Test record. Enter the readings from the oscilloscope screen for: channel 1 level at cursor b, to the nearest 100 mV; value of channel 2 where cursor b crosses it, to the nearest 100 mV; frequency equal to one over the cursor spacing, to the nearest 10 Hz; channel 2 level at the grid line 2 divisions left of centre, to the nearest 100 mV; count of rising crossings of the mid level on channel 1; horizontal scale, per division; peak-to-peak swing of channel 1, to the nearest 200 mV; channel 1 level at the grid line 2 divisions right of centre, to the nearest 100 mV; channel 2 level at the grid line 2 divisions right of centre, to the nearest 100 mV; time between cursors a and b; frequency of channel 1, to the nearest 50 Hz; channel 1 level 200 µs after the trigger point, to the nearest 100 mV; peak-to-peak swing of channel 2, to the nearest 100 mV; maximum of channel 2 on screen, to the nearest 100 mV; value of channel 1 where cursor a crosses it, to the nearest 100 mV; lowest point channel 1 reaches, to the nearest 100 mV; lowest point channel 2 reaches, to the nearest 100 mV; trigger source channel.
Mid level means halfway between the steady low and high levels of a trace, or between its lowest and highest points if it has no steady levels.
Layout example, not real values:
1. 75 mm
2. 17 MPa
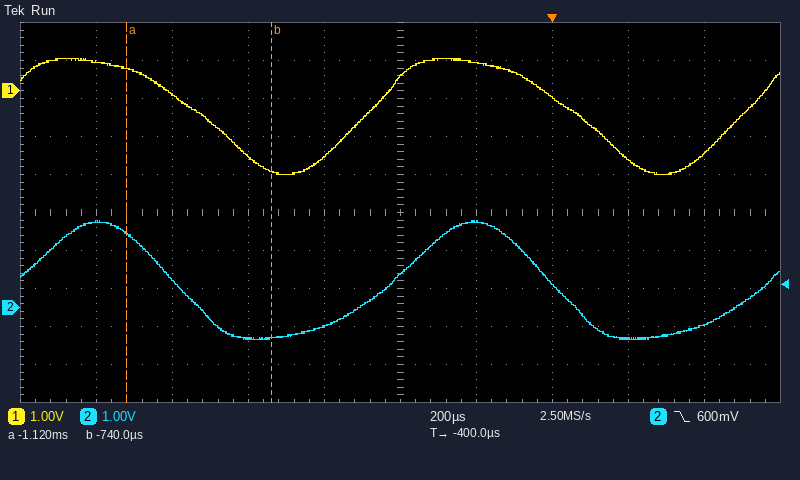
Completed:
1. -2.1 V
2. -800 mV
3. 2.63 kHz
4. -800 mV
5. 2
6. 200 µs
7. 3.0 V
8. -200 mV
9. 600 mV
10. 380 µs
11. 1.00 kHz
12. -1.8 V
13. 3.1 V
14. 2.3 V
15. 600 mV
16. -2.2 V
17. -800 mV
18. channel 2
